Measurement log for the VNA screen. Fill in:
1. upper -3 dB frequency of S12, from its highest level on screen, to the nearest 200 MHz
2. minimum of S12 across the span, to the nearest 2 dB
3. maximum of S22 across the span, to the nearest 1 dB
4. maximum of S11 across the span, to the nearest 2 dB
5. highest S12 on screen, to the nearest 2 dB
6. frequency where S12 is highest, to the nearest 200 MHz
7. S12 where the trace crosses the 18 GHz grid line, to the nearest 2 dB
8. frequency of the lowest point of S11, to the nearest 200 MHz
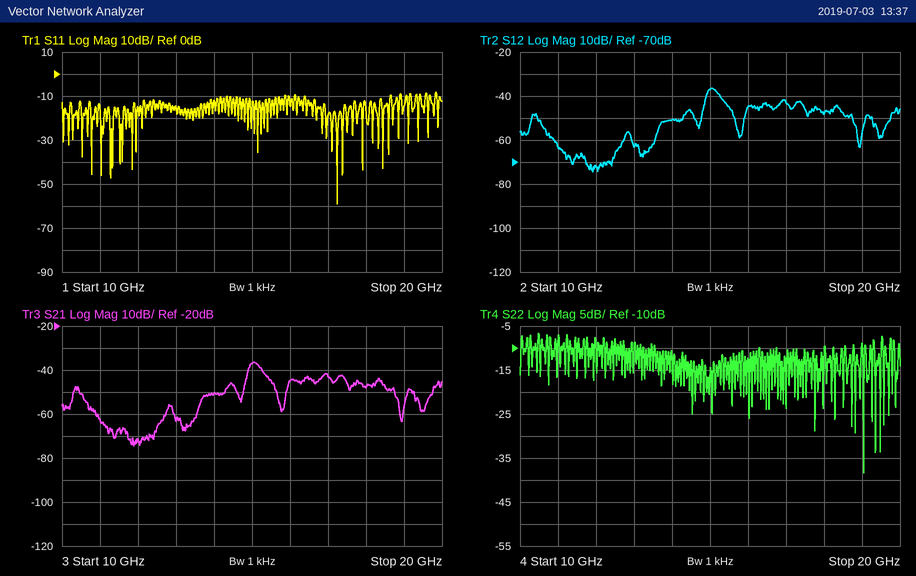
15.2 GHz
-74 dB
-7 dB
-8 dB
-36 dB
15.0 GHz
-48 dB
17.2 GHz
